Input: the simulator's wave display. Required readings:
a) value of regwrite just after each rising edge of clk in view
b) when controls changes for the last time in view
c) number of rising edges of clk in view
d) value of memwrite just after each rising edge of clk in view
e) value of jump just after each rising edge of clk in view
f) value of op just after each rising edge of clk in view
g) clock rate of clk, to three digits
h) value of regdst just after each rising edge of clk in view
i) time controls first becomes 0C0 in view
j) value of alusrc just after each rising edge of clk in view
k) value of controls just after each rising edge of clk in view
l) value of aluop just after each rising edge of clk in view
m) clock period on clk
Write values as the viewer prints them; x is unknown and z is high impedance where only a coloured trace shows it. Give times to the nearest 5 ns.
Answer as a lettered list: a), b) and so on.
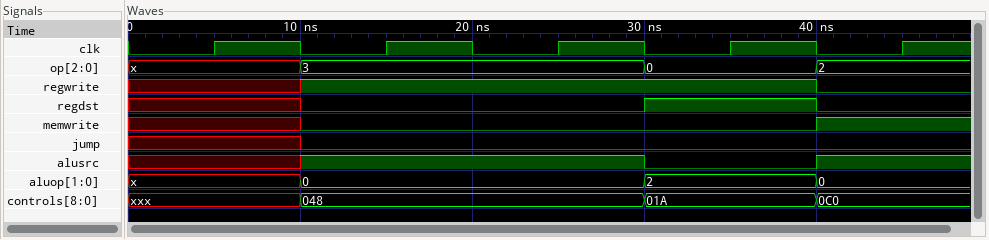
a) x 1 1 1 0
b) 40 ns
c) 5
d) x 0 0 0 1
e) x 0 0 0 0
f) x, 3, 3, 0, 2
g) 100 MHz
h) x 0 0 1 0
i) 40 ns
j) x 1 1 0 1
k) xxx, 048, 048, 01A, 0C0
l) x, 0, 0, 2, 0
m) 10 ns
